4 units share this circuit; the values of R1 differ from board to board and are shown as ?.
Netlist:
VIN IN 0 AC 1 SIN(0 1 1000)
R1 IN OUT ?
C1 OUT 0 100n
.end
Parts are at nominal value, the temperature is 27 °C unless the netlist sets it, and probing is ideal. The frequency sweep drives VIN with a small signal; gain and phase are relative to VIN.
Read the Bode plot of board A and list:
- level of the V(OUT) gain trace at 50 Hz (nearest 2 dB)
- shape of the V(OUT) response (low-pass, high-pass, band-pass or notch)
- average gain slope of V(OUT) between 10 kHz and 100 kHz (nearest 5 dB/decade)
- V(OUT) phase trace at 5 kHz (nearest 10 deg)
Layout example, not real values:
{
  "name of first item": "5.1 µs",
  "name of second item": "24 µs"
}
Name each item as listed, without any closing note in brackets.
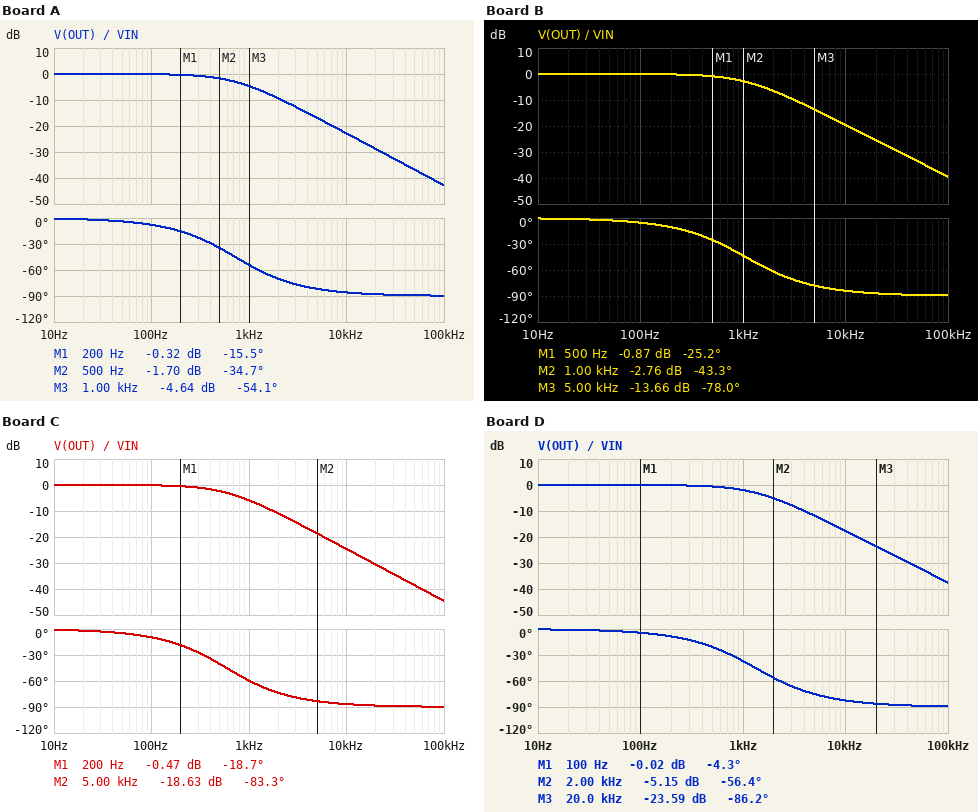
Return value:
{
  "level of the V(OUT) gain trace at 50 Hz": "0 dB",
  "shape of the V(OUT) response": "low-pass",
  "average gain slope of V(OUT) between 10 kHz and 100 kHz": "-20 dB/decade",
  "V(OUT) phase trace at 5 kHz": "-80 deg"
}
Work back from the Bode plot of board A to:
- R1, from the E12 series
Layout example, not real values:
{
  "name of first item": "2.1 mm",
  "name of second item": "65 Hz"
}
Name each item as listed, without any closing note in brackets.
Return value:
{
  "R1, from the E12 series": "2.2 kΩ"
}
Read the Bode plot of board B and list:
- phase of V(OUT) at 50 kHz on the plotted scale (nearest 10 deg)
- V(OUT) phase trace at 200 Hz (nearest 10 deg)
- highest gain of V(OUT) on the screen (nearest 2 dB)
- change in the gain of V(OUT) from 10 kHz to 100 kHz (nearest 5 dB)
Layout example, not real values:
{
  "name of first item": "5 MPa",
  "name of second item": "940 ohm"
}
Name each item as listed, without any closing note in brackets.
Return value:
{
  "phase of V(OUT) at 50 kHz on the plotted scale": "-90 deg",
  "V(OUT) phase trace at 200 Hz": "-10 deg",
  "highest gain of V(OUT) on the screen": "0 dB",
  "change in the gain of V(OUT) from 10 kHz to 100 kHz": "-20 dB"
}
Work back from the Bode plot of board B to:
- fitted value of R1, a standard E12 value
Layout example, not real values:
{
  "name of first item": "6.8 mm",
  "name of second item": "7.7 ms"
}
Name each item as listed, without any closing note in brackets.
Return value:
{
  "fitted value of R1, a standard E12 value": "1.5 kΩ"
}
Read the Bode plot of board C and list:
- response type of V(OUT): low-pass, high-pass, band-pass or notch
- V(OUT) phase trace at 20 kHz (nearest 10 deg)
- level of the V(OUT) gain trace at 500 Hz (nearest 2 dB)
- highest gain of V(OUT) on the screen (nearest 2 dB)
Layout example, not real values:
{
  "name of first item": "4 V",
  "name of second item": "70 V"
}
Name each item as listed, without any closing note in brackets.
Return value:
{
  "response type of V(OUT): low-pass, high-pass, band-pass or notch": "low-pass",
  "V(OUT) phase trace at 20 kHz": "-90 deg",
  "level of the V(OUT) gain trace at 500 Hz": "-2 dB",
  "highest gain of V(OUT) on the screen": "0 dB"
}
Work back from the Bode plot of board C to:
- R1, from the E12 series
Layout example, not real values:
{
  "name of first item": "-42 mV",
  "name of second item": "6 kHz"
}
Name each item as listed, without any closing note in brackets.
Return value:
{
  "R1, from the E12 series": "2.7 kΩ"
}
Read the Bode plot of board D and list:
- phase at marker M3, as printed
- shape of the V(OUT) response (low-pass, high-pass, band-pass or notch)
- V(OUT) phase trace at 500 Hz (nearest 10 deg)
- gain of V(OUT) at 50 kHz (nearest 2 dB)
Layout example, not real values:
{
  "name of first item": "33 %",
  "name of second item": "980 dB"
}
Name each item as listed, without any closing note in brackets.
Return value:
{
  "phase at marker M3, as printed": "-86.2 deg",
  "shape of the V(OUT) response": "low-pass",
  "V(OUT) phase trace at 500 Hz": "-20 deg",
  "gain of V(OUT) at 50 kHz": "-32 dB"
}
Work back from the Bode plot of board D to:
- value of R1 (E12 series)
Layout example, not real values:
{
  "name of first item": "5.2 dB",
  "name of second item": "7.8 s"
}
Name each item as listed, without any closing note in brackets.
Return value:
{
  "value of R1": "1.2 kΩ"
}
